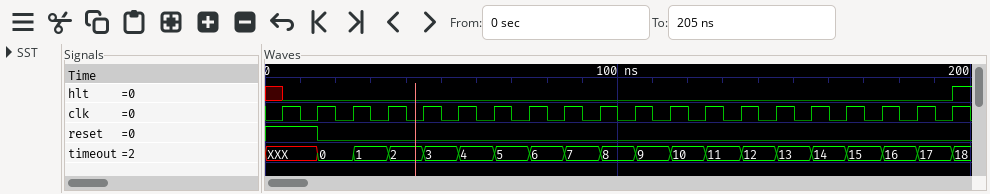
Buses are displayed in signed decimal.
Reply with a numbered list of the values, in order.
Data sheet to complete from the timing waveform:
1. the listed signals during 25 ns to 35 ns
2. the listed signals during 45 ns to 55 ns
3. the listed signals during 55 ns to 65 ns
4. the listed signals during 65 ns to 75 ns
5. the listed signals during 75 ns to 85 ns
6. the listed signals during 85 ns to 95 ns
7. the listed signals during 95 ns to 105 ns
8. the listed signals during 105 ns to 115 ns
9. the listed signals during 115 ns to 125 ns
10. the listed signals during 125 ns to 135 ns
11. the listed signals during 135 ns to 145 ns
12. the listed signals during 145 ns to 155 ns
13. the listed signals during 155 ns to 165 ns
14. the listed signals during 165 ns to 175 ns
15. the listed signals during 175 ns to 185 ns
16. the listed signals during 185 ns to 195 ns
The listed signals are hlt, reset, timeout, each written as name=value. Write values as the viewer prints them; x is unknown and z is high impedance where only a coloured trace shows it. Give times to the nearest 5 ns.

1. hlt=0, reset=0, timeout=1
2. hlt=0, reset=0, timeout=3
3. hlt=0, reset=0, timeout=4
4. hlt=0, reset=0, timeout=5
5. hlt=0, reset=0, timeout=6
6. hlt=0, reset=0, timeout=7
7. hlt=0, reset=0, timeout=8
8. hlt=0, reset=0, timeout=9
9. hlt=0, reset=0, timeout=10
10. hlt=0, reset=0, timeout=11
11. hlt=0, reset=0, timeout=12
12. hlt=0, reset=0, timeout=13
13. hlt=0, reset=0, timeout=14
14. hlt=0, reset=0, timeout=15
15. hlt=0, reset=0, timeout=16
16. hlt=0, reset=0, timeout=17
